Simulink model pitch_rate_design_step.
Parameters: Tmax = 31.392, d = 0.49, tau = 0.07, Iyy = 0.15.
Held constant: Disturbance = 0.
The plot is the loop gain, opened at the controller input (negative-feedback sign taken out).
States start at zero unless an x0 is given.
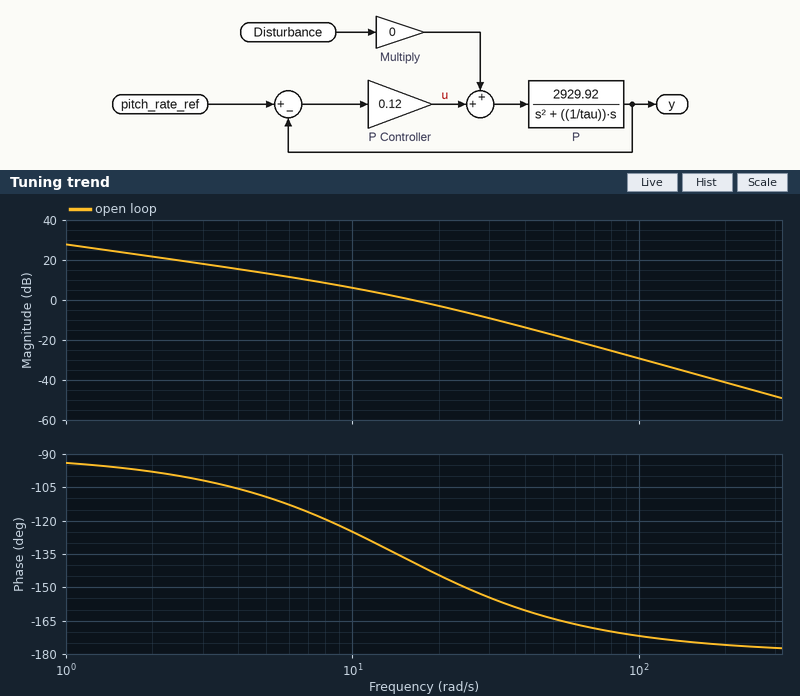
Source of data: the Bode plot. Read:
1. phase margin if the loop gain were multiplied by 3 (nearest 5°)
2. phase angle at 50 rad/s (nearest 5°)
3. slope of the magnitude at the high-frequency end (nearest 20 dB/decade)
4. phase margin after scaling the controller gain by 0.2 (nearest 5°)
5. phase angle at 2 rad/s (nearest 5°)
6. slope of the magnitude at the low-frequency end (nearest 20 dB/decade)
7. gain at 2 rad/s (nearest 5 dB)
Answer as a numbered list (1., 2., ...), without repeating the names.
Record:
1. 25°
2. -165°
3. -40 dB/decade
4. 70°
5. -100°
6. -20 dB/decade
7. 20 dB
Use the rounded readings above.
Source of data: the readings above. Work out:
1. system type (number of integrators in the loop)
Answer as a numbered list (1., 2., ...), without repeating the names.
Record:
1. 1
